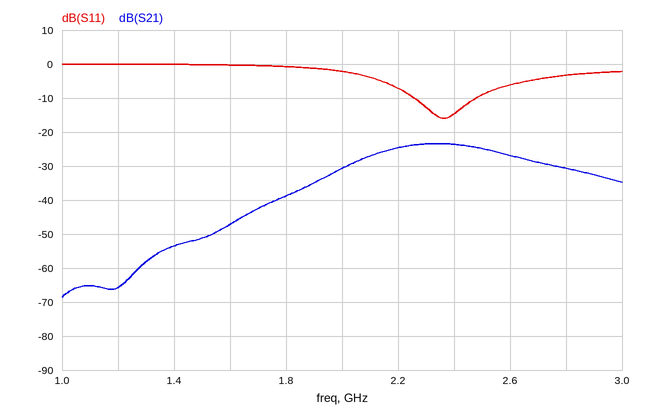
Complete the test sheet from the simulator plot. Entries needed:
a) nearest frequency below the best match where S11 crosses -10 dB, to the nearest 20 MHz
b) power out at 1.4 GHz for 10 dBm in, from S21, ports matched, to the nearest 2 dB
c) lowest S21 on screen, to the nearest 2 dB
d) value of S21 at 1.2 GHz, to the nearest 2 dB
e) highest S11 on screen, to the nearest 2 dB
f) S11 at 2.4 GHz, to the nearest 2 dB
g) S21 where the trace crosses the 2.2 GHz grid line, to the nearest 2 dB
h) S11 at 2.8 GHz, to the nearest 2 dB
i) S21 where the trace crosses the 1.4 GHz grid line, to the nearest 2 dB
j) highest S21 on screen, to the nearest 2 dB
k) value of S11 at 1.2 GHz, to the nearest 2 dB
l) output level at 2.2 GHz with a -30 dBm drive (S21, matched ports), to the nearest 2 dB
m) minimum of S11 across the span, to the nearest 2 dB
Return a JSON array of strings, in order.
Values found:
["2.26 GHz", "-44 dBm", "-68 dB", "-66 dB", "0 dB", "-14 dB", "-24 dB", "-4 dB", "-54 dB", "-24 dB", "0 dB", "-54 dBm", "-16 dB"]
